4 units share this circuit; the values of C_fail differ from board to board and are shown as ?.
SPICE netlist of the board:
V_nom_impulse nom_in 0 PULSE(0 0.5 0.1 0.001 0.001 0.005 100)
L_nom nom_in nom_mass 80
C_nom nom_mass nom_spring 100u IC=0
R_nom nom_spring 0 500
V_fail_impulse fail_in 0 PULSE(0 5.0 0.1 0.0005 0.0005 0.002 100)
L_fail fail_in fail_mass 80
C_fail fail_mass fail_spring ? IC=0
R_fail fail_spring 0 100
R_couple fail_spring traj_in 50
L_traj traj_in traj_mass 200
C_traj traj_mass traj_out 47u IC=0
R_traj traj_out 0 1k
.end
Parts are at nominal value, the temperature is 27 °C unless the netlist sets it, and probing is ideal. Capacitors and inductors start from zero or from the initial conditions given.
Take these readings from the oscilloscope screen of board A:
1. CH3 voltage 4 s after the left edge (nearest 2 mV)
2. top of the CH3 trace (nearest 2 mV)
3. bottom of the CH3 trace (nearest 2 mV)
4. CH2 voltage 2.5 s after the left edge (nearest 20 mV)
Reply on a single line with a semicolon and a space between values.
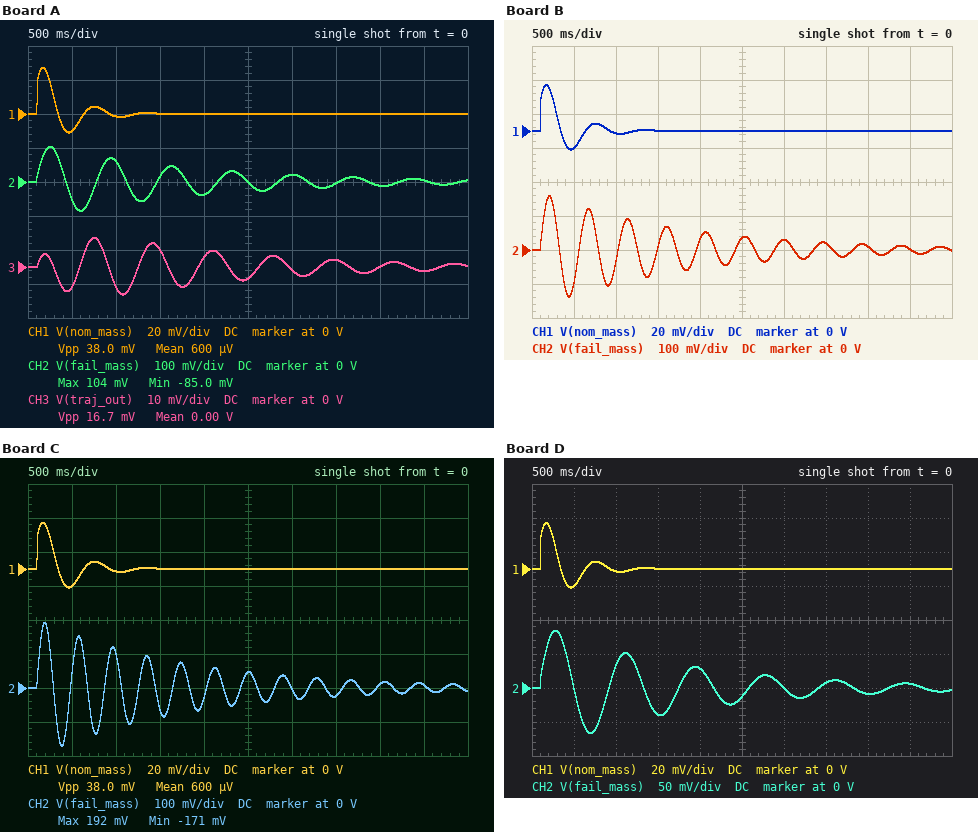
0 V; 8 mV; -8 mV; 0 V
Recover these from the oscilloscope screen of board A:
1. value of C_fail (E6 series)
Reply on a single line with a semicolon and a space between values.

150 µF
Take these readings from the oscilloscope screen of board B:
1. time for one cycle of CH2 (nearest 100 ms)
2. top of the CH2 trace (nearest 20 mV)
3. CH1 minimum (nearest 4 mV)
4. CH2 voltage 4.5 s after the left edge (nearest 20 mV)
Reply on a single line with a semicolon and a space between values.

500 ms; 160 mV; -12 mV; 0 V
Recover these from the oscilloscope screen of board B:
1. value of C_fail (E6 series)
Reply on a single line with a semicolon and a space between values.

68 µF
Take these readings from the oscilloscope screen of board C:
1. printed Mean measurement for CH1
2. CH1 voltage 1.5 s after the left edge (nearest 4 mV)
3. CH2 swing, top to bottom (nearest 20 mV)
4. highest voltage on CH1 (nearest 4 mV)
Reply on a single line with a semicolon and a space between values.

600 µV; 0 V; 360 mV; 28 mV
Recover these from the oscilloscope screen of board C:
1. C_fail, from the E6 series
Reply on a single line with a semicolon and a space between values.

47 µF
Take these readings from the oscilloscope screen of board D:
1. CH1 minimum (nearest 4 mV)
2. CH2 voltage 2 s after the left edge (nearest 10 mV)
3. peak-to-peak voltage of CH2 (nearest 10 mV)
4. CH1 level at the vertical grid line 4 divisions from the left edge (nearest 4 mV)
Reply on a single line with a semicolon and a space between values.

-12 mV; 30 mV; 150 mV; 0 V
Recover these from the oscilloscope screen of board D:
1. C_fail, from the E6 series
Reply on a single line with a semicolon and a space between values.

220 µF
